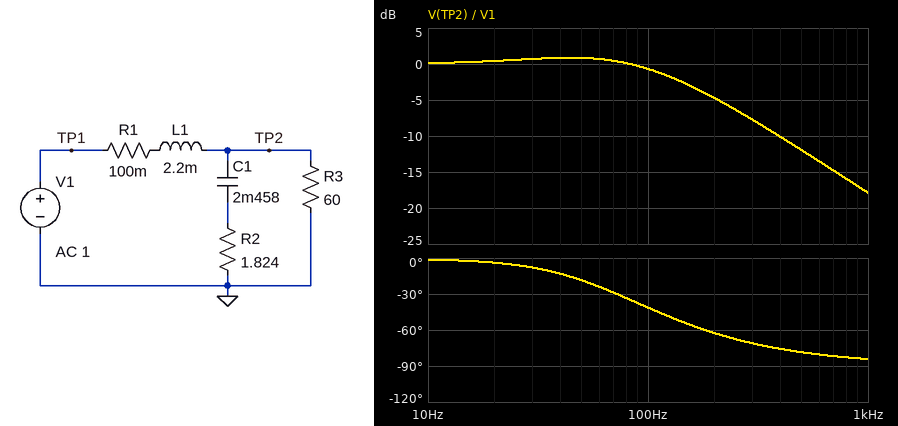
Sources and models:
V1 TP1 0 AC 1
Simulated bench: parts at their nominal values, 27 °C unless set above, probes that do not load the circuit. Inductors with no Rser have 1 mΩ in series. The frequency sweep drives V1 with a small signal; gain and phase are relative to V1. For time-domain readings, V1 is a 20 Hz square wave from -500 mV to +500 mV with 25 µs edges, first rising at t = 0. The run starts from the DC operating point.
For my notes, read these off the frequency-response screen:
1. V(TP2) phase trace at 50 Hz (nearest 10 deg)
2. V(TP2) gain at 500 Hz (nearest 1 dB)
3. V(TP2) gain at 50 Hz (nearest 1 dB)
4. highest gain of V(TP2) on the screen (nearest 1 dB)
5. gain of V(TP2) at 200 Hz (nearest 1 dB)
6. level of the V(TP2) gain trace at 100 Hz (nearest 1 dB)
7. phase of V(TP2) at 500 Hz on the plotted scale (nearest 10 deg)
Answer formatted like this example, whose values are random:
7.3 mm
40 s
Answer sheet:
-20 deg
-12 dB
1 dB
1 dB
-5 dB
-1 dB
-80 deg
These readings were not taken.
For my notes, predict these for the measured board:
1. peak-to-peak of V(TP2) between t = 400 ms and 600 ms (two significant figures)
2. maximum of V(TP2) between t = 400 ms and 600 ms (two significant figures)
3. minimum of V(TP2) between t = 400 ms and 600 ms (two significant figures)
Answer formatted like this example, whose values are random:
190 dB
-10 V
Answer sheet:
1.2 V
600 mV
-600 mV
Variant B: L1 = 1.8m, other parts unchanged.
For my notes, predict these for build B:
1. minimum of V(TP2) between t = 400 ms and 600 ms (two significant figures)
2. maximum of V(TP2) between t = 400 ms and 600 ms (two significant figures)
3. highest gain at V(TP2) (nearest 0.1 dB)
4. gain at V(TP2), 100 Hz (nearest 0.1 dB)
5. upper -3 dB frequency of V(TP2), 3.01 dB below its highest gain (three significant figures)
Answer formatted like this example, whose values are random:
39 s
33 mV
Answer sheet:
-580 mV
580 mV
0.7 dB
-0.3 dB
161 Hz
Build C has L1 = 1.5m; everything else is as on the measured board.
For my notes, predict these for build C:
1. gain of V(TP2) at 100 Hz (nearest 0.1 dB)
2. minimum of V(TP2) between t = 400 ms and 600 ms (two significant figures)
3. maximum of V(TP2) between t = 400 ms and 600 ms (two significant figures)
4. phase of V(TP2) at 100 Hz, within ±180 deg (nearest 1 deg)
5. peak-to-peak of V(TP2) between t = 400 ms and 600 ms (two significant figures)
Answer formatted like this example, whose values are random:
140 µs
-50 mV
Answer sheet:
-0.1 dB
-570 mV
570 mV
-29 deg
1.1 V
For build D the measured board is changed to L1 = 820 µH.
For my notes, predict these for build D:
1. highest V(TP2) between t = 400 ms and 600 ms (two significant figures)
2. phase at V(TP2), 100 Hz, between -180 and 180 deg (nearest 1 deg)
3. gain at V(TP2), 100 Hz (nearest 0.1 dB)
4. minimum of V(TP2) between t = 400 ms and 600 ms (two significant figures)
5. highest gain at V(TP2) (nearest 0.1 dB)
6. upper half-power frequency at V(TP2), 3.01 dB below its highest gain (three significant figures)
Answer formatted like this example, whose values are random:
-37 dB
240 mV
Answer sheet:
530 mV
-16 deg
0 dB
-530 mV
0.2 dB
346 Hz
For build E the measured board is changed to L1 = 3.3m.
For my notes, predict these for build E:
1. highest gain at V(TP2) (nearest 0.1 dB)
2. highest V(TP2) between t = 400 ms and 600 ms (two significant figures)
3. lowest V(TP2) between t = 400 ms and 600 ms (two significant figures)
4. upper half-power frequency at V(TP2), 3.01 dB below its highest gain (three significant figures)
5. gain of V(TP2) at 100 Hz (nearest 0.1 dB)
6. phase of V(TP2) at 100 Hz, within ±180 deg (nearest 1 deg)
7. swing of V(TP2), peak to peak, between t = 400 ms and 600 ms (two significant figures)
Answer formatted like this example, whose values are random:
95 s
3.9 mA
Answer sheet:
1.3 dB
640 mV
-640 mV
94.8 Hz
-2.1 dB
-57 deg
1.3 V
